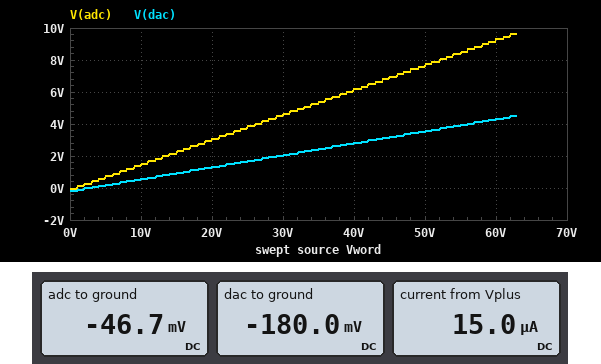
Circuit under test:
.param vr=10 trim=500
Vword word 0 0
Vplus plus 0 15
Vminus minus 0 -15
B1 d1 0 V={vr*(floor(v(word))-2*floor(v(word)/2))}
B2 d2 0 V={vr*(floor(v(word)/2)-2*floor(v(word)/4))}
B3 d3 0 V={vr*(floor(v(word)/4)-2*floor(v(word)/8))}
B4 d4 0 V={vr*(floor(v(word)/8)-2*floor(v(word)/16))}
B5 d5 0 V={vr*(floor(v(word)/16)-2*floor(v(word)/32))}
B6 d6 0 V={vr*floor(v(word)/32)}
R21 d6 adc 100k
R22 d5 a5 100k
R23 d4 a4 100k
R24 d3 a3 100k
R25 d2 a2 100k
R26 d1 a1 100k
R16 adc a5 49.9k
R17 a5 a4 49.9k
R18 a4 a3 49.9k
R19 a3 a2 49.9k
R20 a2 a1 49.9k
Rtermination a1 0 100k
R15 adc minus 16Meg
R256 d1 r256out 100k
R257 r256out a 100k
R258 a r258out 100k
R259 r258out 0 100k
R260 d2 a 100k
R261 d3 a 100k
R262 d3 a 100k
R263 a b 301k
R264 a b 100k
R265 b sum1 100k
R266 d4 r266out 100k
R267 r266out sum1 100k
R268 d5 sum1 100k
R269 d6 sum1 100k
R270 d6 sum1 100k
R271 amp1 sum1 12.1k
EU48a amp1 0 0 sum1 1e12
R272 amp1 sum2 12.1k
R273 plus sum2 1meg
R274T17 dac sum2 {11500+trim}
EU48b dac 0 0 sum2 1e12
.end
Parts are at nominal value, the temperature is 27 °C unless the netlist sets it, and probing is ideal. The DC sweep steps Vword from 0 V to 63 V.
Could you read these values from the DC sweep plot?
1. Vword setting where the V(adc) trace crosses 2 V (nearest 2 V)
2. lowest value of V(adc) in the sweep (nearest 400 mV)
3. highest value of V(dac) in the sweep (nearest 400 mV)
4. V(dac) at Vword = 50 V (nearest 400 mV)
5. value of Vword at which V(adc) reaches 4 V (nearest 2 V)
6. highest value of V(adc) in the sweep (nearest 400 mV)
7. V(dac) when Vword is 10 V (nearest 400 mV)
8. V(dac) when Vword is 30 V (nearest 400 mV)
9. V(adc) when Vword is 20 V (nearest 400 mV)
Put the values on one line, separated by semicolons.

14 V; 0 V; 4.4 V; 3.6 V; 26 V; 9.6 V; 400 mV; 2.0 V; 3.2 V
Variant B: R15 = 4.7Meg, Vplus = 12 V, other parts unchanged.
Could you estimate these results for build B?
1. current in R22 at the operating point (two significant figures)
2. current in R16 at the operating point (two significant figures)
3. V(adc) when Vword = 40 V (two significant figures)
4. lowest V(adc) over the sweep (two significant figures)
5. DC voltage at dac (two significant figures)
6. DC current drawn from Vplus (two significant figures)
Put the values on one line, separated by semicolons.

790 nA; 1.6 µA; 6.0 V; -160 mV; -140 mV; 12 µA
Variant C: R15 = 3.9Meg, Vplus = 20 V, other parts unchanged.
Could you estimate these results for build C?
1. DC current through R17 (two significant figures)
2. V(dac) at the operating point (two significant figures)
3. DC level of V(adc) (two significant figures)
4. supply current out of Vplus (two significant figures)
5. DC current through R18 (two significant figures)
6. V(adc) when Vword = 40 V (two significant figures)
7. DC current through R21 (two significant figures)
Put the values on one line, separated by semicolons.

950 nA; -240 mV; -190 mV; 20 µA; 480 nA; 6.0 V; 1.9 µA
